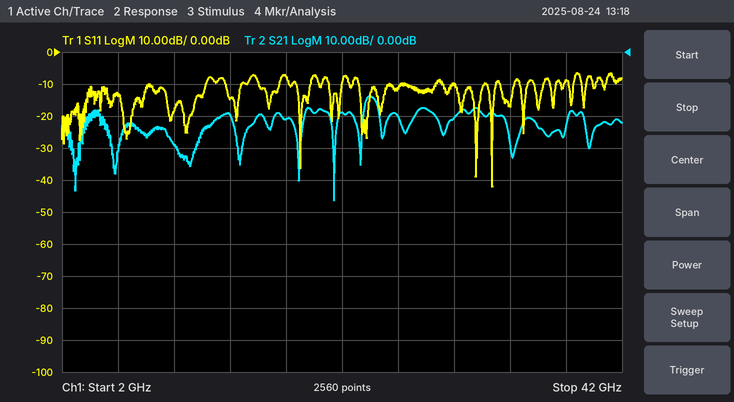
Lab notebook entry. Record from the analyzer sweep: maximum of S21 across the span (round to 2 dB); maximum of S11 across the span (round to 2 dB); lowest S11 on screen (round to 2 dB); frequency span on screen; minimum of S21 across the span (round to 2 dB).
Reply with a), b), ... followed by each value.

a) -14 dB
b) -6 dB
c) -42 dB
d) 40 GHz
e) -46 dB
